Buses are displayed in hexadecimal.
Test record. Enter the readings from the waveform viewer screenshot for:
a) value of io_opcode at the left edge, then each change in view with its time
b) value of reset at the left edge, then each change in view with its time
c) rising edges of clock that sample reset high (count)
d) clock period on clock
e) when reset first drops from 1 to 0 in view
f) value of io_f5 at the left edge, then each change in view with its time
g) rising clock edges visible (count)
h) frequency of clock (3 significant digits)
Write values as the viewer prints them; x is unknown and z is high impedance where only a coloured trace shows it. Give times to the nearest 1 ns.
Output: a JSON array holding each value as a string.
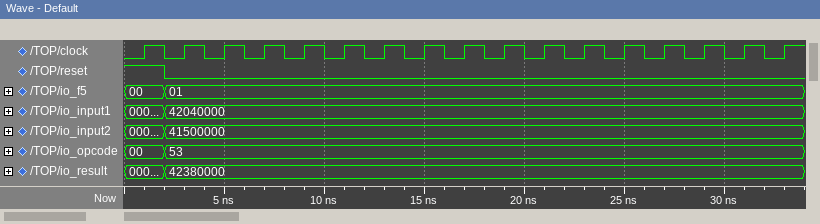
["00, 53 at 2 ns", "1, 0 at 2 ns", "1", "2 ns", "2 ns", "00, 01 at 2 ns", "17", "500 MHz"]
